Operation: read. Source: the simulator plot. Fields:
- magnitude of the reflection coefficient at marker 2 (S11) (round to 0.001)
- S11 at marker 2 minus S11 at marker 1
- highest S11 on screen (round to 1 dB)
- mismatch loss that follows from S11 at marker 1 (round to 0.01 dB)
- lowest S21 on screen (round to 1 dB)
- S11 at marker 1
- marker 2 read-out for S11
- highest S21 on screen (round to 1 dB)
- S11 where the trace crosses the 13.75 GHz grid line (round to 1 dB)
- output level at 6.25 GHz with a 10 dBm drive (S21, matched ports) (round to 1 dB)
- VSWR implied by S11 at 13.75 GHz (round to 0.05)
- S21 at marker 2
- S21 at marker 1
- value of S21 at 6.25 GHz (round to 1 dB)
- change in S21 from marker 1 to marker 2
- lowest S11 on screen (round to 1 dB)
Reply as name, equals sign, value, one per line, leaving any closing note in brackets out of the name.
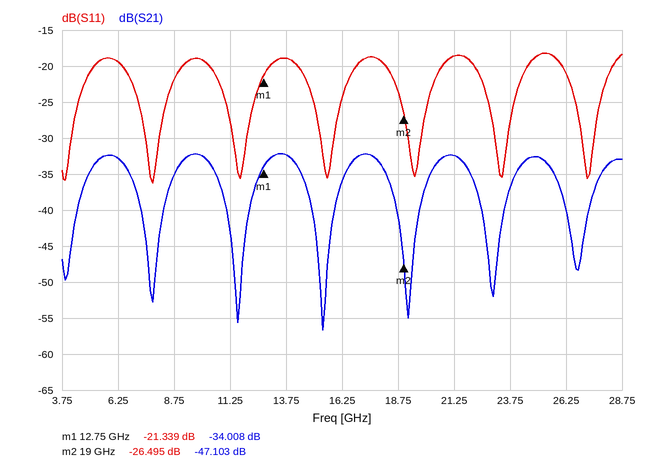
magnitude of the reflection coefficient at marker 2 (S11) = 0.047
S11 at marker 2 minus S11 at marker 1 = -5.156 dB
highest S11 on screen = -18 dB
mismatch loss that follows from S11 at marker 1 = 0.03 dB
lowest S21 on screen = -57 dB
S11 at marker 1 = -21.339 dB
marker 2 read-out for S11 = -26.495 dB
highest S21 on screen = -32 dB
S11 where the trace crosses the 13.75 GHz grid line = -19 dB
output level at 6.25 GHz with a 10 dBm drive (S21, matched ports) = -23 dBm
VSWR implied by S11 at 13.75 GHz = 1.25
S21 at marker 2 = -47.103 dB
S21 at marker 1 = -34.008 dB
value of S21 at 6.25 GHz = -33 dB
change in S21 from marker 1 to marker 2 = -13.095 dB
lowest S11 on screen = -36 dB
